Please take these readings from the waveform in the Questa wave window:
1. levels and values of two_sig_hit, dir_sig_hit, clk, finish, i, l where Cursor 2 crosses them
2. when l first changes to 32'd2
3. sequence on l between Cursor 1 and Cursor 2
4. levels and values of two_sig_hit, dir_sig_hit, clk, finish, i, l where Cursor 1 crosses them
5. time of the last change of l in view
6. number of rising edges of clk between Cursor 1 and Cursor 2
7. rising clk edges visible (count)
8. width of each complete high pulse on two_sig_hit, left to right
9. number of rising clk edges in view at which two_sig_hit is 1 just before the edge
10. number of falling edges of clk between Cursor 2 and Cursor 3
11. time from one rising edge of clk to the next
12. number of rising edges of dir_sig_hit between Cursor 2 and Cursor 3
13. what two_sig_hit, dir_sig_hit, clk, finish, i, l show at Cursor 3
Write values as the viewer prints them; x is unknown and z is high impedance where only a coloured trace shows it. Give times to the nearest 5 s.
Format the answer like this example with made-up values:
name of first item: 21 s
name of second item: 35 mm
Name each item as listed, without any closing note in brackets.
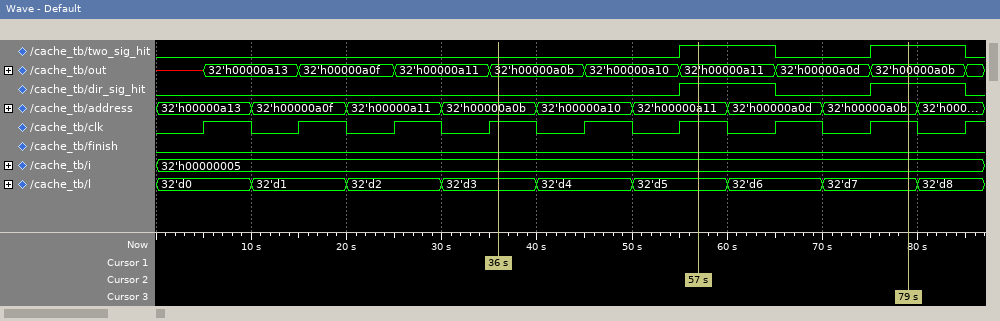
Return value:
levels and values of two_sig_hit, dir_sig_hit, clk, finish, i, l where Cursor 2 crosses them: two_sig_hit=1, dir_sig_hit=1, clk=1, finish=0, i=32'h00000005, l=32'd5
when l first changes to 32'd2: 20 s
sequence on l between Cursor 1 and Cursor 2: 32'd3, 32'd4, 32'd5
levels and values of two_sig_hit, dir_sig_hit, clk, finish, i, l where Cursor 1 crosses them: two_sig_hit=0, dir_sig_hit=0, clk=1, finish=0, i=32'h00000005, l=32'd3
time of the last change of l in view: 80 s
number of rising edges of clk between Cursor 1 and Cursor 2: 2
rising clk edges visible: 9
width of each complete high pulse on two_sig_hit, left to right: 10 s, 10 s
number of rising clk edges in view at which two_sig_hit is 1 just before the edge: 2
number of falling edges of clk between Cursor 2 and Cursor 3: 2
time from one rising edge of clk to the next: 10 s
number of rising edges of dir_sig_hit between Cursor 2 and Cursor 3: 1
what two_sig_hit, dir_sig_hit, clk, finish, i, l show at Cursor 3: two_sig_hit=1, dir_sig_hit=1, clk=1, finish=0, i=32'h00000005, l=32'd7
